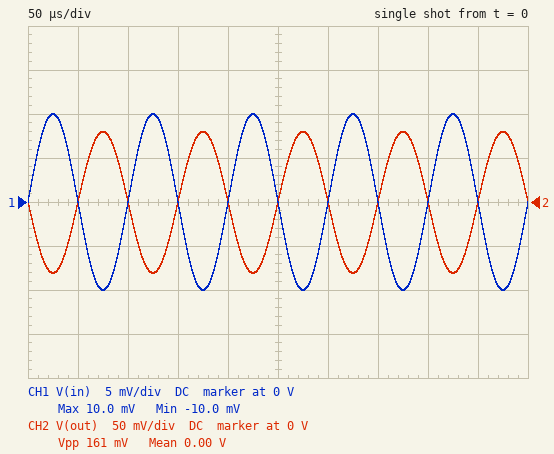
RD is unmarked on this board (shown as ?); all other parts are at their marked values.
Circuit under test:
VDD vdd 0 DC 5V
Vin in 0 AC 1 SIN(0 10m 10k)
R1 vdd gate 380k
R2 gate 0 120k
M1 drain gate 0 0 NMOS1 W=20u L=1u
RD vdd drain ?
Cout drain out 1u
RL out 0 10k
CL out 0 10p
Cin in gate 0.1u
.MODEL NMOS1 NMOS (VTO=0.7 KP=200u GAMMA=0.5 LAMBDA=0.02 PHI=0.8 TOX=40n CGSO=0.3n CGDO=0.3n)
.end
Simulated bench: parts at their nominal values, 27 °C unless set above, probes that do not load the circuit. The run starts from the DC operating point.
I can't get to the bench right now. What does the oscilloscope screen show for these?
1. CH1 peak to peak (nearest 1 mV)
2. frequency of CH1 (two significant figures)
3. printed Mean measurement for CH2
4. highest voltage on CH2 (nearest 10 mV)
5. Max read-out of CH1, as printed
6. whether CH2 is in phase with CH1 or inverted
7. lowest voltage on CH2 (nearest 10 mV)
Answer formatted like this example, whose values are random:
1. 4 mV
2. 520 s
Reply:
1. 20 mV
2. 10 kHz
3. 0.00 V
4. 80 mV
5. 10.0 mV
6. inverted
7. -80 mV
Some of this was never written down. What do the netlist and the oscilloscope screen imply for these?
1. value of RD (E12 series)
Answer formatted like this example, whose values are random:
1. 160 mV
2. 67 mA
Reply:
1. 6.8 kΩ
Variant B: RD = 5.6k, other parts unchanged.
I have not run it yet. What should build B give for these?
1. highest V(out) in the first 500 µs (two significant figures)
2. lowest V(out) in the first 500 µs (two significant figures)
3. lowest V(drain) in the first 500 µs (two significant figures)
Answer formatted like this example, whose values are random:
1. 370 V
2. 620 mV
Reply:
1. 72 mV
2. -73 mV
3. 2.0 V
